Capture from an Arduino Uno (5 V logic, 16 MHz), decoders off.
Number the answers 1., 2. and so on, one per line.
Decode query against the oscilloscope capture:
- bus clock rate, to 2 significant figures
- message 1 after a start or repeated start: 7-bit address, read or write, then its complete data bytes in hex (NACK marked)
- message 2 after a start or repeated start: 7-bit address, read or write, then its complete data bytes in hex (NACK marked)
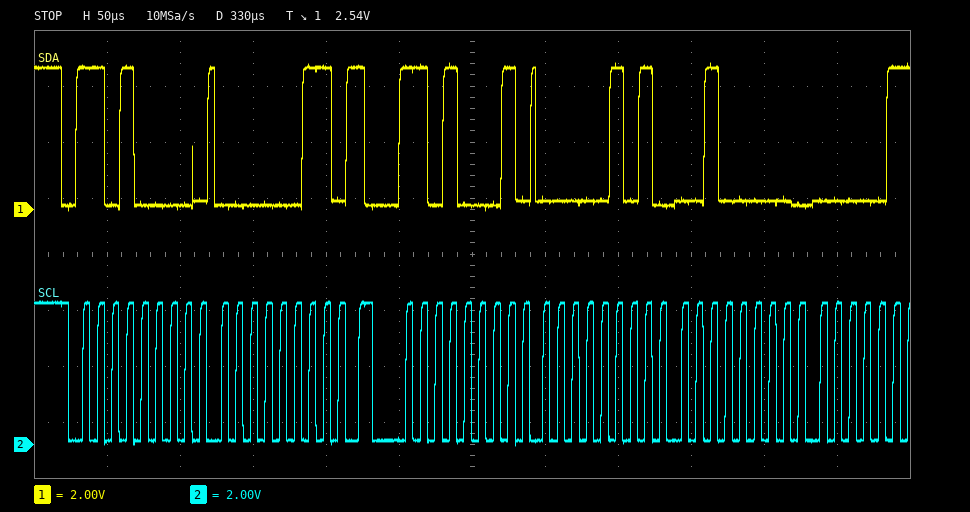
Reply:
1. 100 kHz
2. 0x68 write: 03
3. 0x68 read: 05 20
